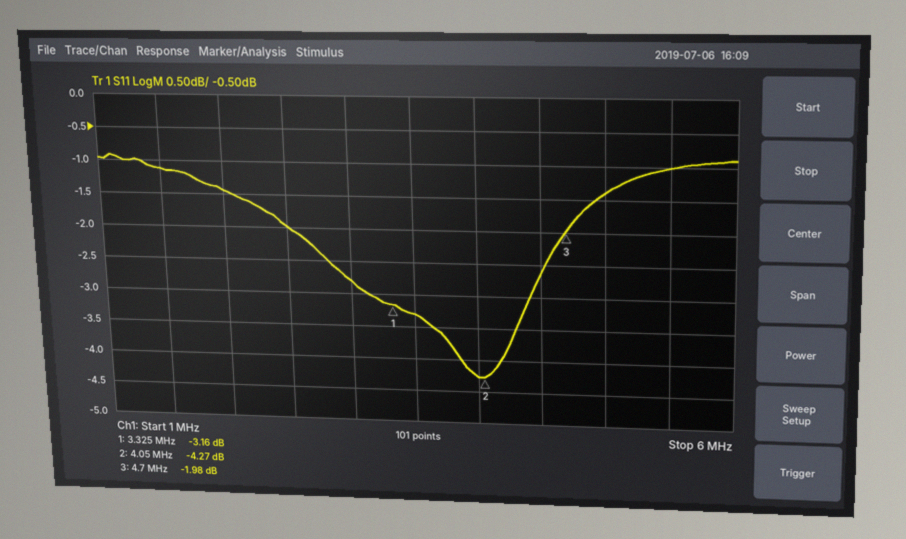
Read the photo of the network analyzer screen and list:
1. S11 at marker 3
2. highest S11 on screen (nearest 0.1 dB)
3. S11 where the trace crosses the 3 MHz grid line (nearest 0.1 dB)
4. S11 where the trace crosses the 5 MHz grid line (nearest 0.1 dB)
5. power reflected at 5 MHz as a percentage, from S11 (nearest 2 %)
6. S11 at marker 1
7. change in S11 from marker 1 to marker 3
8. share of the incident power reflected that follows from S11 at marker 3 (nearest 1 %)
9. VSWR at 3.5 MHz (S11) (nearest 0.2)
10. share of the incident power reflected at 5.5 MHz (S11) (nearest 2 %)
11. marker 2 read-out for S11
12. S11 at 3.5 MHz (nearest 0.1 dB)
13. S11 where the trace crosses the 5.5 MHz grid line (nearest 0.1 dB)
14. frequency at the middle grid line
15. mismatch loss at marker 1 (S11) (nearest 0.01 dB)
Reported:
-1.98 dB
-0.9 dB
-2.8 dB
-1.4 dB
72 %
-3.16 dB
1.18 dB
63 %
5.4
80 %
-4.27 dB
-3.3 dB
-1.0 dB
3.5 MHz
2.87 dB
